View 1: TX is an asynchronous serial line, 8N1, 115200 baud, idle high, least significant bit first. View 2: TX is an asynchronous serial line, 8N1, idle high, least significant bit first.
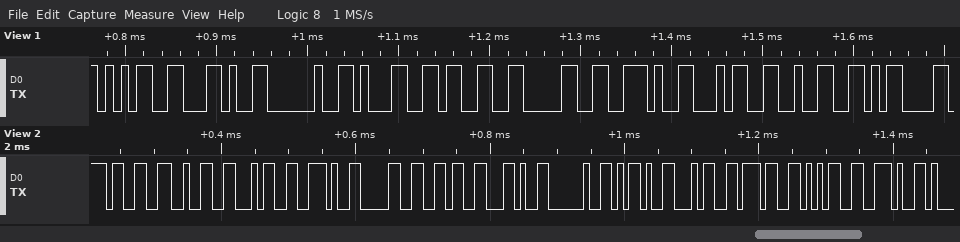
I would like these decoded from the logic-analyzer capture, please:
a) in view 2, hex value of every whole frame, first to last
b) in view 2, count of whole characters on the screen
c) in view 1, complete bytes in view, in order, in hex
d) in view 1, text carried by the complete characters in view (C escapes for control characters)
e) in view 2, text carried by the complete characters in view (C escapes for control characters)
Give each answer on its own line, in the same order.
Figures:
33 32 34 2E 30 36 2C 20 2D 34 37 35 2E
13
35 2C 20 31 33 30 2E 34 32 0D
"5, 130.42\r"
"324.06, -475."
